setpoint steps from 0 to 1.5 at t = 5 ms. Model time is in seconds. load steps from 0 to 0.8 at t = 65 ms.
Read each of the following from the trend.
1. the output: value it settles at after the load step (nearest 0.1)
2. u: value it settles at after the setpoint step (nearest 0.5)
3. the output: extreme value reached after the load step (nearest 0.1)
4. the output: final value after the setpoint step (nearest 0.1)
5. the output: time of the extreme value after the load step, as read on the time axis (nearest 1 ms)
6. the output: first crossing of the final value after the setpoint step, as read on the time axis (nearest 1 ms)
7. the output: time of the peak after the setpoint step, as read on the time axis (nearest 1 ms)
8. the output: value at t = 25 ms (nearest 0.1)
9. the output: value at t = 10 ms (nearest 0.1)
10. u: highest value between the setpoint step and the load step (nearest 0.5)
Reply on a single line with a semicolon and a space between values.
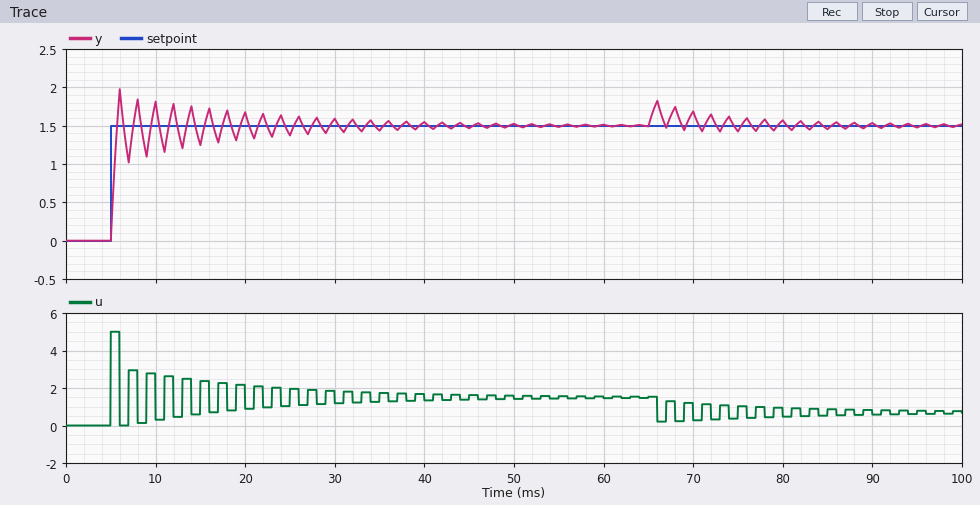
1.5; 1.5; 1.8; 1.5; 66 ms; 6 ms; 6 ms; 1.4; 1.8; 5.0
